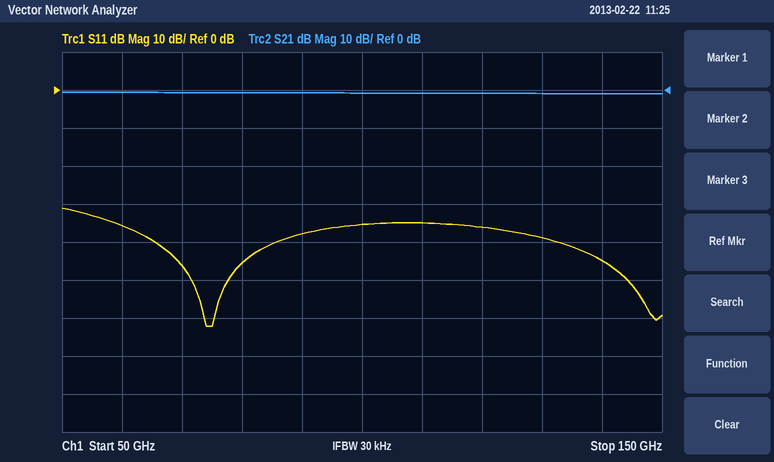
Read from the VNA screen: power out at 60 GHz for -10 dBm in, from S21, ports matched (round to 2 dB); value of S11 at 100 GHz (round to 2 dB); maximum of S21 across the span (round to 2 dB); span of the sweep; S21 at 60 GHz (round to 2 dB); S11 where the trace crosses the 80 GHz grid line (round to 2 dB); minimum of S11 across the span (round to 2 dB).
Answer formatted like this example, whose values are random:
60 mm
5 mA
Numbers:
-10 dBm
-36 dB
0 dB
100 GHz
0 dB
-46 dB
-62 dB
